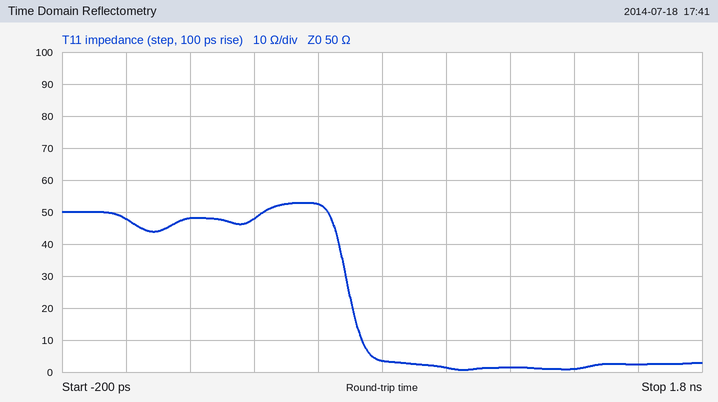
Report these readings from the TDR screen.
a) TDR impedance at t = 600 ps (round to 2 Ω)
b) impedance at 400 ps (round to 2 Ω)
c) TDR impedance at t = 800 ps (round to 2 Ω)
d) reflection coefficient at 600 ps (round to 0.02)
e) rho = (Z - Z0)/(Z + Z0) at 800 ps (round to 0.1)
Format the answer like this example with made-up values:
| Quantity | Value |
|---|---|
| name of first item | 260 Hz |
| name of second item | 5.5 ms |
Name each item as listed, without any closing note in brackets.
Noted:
| Quantity | Value |
|---|---|
| TDR impedance at t = 600 ps | 52 Ω |
| impedance at 400 ps | 48 Ω |
| TDR impedance at t = 800 ps | 4 Ω |
| reflection coefficient at 600 ps | +0.02 |
| rho = (Z - Z0)/(Z + Z0) at 800 ps | -0.9 |
